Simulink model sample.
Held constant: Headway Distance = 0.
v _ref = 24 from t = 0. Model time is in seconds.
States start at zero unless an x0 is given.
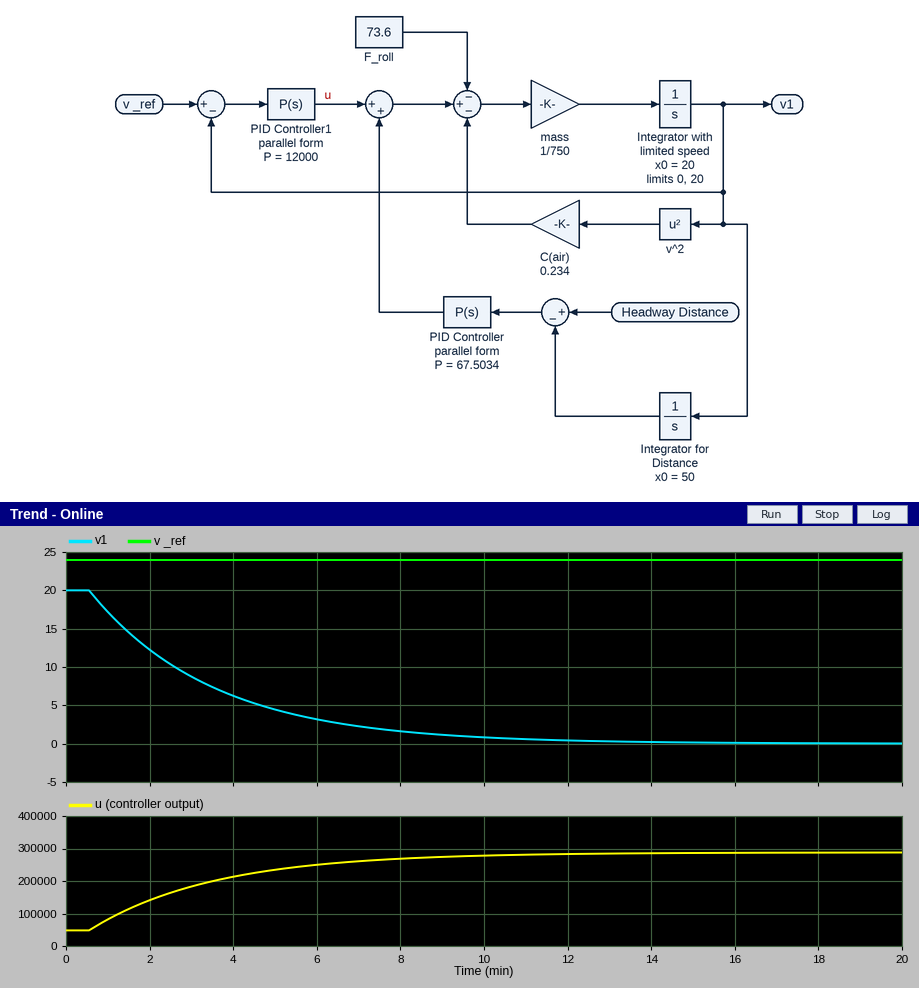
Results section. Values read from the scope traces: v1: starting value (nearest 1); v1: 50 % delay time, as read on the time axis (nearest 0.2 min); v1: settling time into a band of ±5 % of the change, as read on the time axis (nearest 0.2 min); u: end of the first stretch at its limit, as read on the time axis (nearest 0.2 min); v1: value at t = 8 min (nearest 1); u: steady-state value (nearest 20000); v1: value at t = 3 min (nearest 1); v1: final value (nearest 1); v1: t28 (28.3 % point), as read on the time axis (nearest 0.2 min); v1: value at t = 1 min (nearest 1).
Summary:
20
2.6 min
9.4 min
0.6 min
2
280000
9
0
1.6 min
17
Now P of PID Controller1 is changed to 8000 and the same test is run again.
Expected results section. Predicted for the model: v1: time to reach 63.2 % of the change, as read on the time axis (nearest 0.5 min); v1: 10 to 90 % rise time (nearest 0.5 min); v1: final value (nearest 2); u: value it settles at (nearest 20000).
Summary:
2.5 min
4.5 min
0
200000
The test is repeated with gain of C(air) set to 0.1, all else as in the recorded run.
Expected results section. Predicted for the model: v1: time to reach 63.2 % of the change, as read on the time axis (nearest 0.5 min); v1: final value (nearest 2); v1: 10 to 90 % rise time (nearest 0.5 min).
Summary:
3.5 min
0
6.5 min
